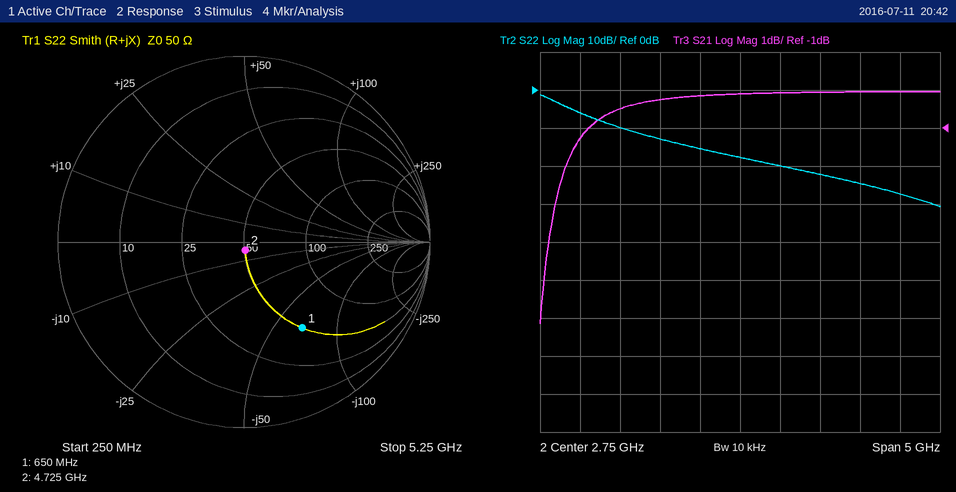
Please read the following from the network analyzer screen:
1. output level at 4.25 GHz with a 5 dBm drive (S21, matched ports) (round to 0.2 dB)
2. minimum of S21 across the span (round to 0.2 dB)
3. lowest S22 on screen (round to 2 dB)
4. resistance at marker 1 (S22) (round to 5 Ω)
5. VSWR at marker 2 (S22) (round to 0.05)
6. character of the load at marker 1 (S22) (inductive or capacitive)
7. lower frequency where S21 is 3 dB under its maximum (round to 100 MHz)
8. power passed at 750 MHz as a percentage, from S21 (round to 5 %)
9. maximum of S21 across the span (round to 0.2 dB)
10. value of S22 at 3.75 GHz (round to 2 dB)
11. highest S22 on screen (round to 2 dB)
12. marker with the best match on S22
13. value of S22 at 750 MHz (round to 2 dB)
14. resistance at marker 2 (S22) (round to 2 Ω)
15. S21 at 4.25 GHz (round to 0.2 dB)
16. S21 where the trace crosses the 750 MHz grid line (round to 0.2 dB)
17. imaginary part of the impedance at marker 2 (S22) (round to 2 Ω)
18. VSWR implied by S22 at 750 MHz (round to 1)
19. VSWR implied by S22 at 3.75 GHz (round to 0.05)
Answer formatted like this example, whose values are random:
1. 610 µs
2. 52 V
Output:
1. 5.0 dBm
2. -6.2 dB
3. -30 dB
4. 50 Ω
5. 1.10
6. capacitive
7. 400 MHz
8. 75 %
9. 0.0 dB
10. -22 dB
11. -2 dB
12. marker 2
13. -6 dB
14. 50 Ω
15. 0.0 dB
16. -1.2 dB
17. -4 Ω
18. 3
19. 1.15
